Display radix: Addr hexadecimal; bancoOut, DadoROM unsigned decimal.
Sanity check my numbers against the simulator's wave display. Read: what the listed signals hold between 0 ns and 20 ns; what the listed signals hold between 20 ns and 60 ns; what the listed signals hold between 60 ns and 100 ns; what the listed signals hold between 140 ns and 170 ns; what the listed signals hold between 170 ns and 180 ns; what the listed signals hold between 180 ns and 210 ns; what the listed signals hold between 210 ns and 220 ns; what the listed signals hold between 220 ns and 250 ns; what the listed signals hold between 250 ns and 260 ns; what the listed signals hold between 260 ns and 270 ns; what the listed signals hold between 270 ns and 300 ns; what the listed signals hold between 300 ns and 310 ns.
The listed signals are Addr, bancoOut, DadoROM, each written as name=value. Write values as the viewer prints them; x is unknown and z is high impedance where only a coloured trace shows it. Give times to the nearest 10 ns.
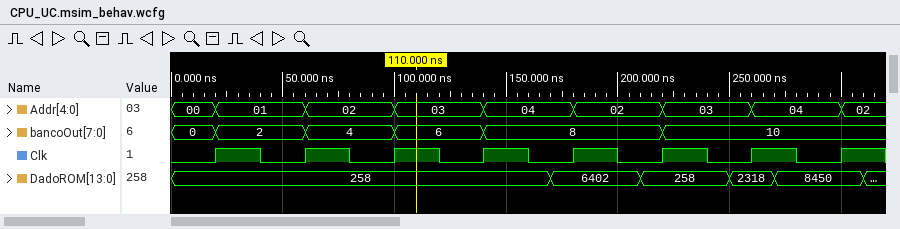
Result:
Addr=00, bancoOut=0, DadoROM=258
Addr=01, bancoOut=2, DadoROM=258
Addr=02, bancoOut=4, DadoROM=258
Addr=04, bancoOut=8, DadoROM=258
Addr=04, bancoOut=8, DadoROM=6402
Addr=02, bancoOut=8, DadoROM=6402
Addr=02, bancoOut=8, DadoROM=258
Addr=03, bancoOut=10, DadoROM=258
Addr=03, bancoOut=10, DadoROM=2318
Addr=04, bancoOut=10, DadoROM=2318
Addr=04, bancoOut=10, DadoROM=8450
Addr=02, bancoOut=10, DadoROM=8450
